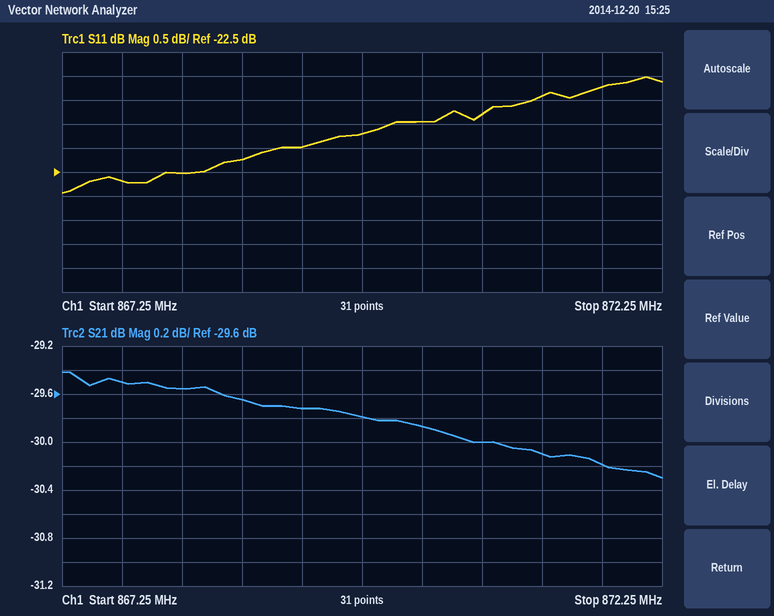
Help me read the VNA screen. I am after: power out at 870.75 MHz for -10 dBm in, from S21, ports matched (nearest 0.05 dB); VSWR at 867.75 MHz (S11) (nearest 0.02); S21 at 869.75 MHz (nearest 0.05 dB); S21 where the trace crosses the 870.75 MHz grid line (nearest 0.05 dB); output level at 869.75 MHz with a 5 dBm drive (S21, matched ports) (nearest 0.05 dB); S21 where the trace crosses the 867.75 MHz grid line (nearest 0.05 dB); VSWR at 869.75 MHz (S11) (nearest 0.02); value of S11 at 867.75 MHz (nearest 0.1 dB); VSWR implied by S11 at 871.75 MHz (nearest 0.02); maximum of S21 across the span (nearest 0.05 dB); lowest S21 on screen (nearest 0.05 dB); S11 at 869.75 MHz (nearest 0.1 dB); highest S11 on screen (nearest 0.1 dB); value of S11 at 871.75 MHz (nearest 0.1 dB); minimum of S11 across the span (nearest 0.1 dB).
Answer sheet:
-40.00 dBm
1.16
-29.80 dB
-30.00 dB
-24.80 dBm
-29.50 dB
1.18
-22.7 dB
1.20
-29.40 dB
-30.30 dB
-21.7 dB
-20.5 dB
-20.7 dB
-22.9 dB
